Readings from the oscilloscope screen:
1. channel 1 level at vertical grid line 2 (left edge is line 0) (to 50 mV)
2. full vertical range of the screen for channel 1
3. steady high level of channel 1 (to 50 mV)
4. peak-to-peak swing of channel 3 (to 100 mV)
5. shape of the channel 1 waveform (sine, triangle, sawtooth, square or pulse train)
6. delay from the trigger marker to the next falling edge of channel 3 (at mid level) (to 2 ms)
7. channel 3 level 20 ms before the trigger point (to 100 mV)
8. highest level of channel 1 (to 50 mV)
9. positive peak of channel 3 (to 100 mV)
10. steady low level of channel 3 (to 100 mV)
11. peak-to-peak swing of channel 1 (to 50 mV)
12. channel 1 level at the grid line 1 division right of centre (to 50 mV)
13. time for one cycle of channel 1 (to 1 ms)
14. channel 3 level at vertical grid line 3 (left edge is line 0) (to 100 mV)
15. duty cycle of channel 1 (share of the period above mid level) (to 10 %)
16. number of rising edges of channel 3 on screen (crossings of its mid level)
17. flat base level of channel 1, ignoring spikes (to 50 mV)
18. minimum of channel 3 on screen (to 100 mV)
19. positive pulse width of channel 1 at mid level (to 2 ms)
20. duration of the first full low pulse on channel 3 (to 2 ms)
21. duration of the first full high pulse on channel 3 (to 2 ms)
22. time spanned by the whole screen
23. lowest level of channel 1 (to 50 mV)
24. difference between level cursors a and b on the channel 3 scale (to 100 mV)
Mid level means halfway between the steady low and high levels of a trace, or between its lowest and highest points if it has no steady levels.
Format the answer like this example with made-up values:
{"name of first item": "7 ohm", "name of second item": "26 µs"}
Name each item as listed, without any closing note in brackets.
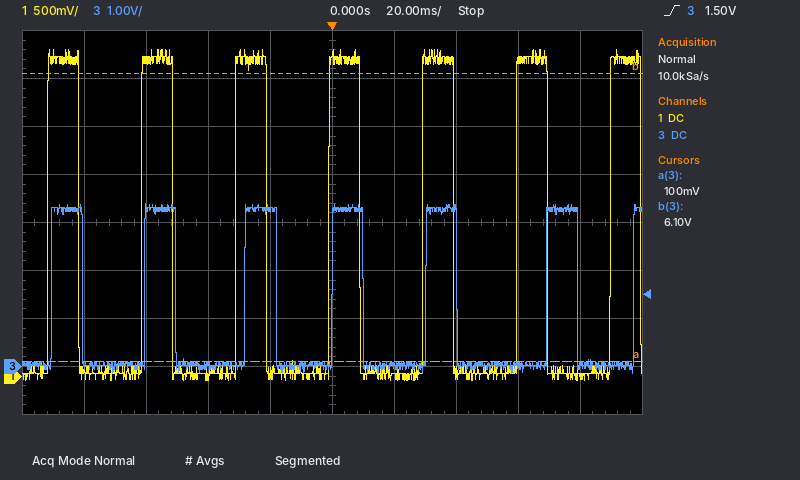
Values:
{"channel 1 level at vertical grid line 2 (left edge is line 0)": "3.30 V", "full vertical range of the screen for channel 1": "4 V", "steady high level of channel 1": "3.30 V", "peak-to-peak swing of channel 3": "3.5 V", "shape of the channel 1 waveform": "pulse train", "delay from the trigger marker to the next falling edge of channel 3 (at mid level)": "10 ms", "channel 3 level 20 ms before the trigger point": "3.3 V", "highest level of channel 1": "3.40 V", "positive peak of channel 3": "3.4 V", "steady low level of channel 3": "0.0 V", "peak-to-peak swing of channel 1": "3.45 V", "channel 1 level at the grid line 1 division right of centre": "0 mV", "time for one cycle of channel 1": "30 ms", "channel 3 level at vertical grid line 3 (left edge is line 0)": "0.0 V", "duty cycle of channel 1 (share of the period above mid level)": "30 %", "number of rising edges of channel 3 on screen": "7", "flat base level of channel 1, ignoring spikes": "50 mV", "minimum of channel 3 on screen": "-100 mV", "positive pulse width of channel 1 at mid level": "10 ms", "duration of the first full low pulse on channel 3": "20 ms", "duration of the first full high pulse on channel 3": "10 ms", "time spanned by the whole screen": "200 ms", "lowest level of channel 1": "-50 mV", "difference between level cursors a and b on the channel 3 scale": "6.0 V"}
